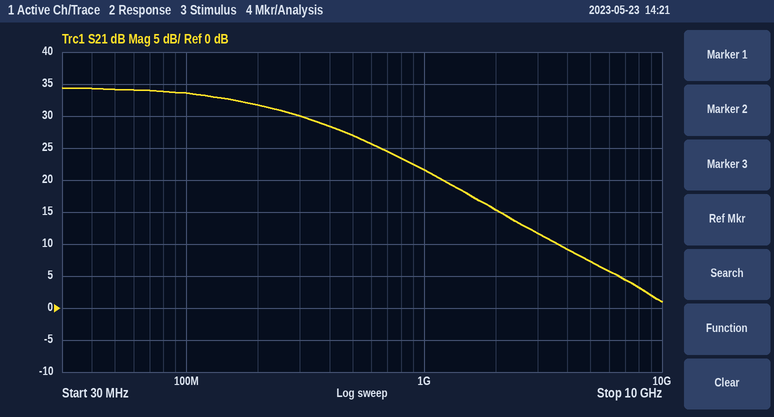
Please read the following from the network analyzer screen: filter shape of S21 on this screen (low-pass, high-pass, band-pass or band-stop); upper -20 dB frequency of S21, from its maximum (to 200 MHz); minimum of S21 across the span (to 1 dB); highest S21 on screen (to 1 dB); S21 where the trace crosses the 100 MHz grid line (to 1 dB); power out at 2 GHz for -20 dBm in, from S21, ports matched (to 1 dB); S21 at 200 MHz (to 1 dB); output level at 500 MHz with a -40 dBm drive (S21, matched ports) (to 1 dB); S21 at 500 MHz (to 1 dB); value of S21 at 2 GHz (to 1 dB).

low-pass
2.2 GHz
1 dB
34 dB
34 dB
-5 dBm
32 dB
-13 dBm
27 dB
15 dB
